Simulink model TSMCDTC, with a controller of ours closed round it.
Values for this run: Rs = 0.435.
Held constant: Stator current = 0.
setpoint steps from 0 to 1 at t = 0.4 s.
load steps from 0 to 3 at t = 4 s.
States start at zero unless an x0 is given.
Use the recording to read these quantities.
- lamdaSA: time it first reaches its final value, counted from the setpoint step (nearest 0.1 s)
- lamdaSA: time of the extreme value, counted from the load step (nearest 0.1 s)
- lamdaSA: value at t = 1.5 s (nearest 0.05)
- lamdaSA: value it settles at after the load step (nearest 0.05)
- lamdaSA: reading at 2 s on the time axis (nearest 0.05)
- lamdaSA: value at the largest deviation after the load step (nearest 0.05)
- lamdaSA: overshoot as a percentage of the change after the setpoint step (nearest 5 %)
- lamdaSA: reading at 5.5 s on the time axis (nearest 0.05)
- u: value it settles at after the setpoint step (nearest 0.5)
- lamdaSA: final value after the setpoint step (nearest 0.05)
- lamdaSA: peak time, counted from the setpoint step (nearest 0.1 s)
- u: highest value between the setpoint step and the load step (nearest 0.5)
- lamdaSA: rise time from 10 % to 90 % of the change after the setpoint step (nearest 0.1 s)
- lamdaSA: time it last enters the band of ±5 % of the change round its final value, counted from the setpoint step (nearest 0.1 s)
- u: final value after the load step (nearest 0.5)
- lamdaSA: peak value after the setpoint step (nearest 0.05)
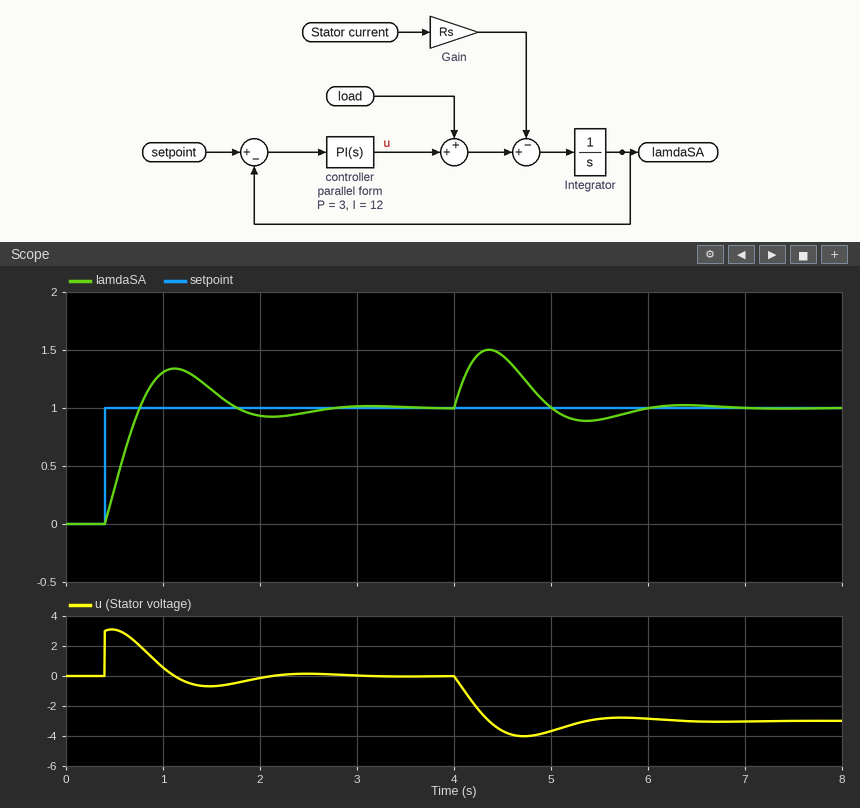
0.4 s
0.4 s
1.15
1.00
0.95
1.50
35 %
0.90
0.0
1.00
0.7 s
3.0
0.3 s
2.0 s
-3.0
1.35
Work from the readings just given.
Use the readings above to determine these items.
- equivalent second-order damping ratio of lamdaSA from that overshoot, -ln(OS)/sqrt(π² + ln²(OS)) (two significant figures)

0.32
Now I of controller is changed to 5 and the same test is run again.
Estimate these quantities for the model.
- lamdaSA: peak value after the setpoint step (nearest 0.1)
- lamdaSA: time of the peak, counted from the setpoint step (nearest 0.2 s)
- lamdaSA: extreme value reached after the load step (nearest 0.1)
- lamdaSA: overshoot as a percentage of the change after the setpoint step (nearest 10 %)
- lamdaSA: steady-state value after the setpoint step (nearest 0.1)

1.2
1.0 s
1.6
20 %
1.0
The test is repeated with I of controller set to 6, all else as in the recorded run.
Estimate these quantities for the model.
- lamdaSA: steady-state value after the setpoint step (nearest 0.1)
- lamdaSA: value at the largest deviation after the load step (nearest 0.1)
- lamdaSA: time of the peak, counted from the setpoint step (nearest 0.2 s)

1.0
1.6
1.0 s
